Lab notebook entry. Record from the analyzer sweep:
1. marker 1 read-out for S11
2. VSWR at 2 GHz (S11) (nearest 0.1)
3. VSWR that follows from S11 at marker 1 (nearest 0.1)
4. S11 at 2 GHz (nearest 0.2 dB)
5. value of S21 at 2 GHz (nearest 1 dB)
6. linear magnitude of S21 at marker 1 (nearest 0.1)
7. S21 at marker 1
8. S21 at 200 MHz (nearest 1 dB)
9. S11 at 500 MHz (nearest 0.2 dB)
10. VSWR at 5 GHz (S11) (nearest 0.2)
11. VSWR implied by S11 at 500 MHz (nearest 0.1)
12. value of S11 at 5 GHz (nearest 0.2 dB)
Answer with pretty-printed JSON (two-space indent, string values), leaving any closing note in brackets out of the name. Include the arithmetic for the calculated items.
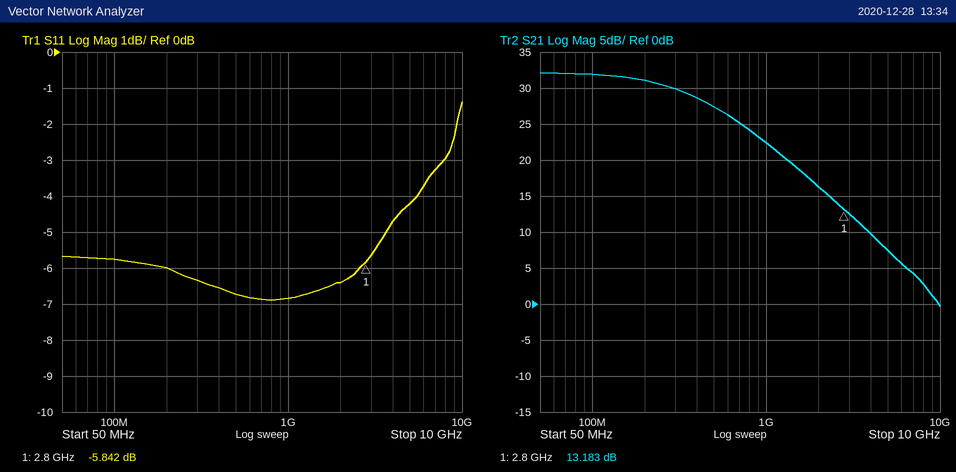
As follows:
{
  "marker 1 read-out for S11": "-5.842 dB",
  "VSWR at 2 GHz (S11)": "|Γ| = 10^(-6.4/20) = 0.4786; VSWR = (1 + 0.4786)/(1 − 0.4786) ≈ 2.8",
  "VSWR that follows from S11 at marker 1": "(1 + 0.5104)/(1 − 0.5104) ≈ 3.1",
  "S11 at 2 GHz": "-6.4 dB",
  "value of S21 at 2 GHz": "16 dB",
  "linear magnitude of S21 at marker 1": "10^(13.183/20) ≈ 4.6",
  "S21 at marker 1": "13.183 dB",
  "S21 at 200 MHz": "31 dB",
  "S11 at 500 MHz": "-6.8 dB",
  "VSWR at 5 GHz (S11)": "|Γ| = 10^(-4.2/20) = 0.6166; VSWR = (1 + 0.6166)/(1 − 0.6166) ≈ 4.2",
  "VSWR implied by S11 at 500 MHz": "|Γ| = 10^(-6.8/20) = 0.4571; VSWR = (1 + 0.4571)/(1 − 0.4571) ≈ 2.7",
  "value of S11 at 5 GHz": "-4.2 dB"
}
